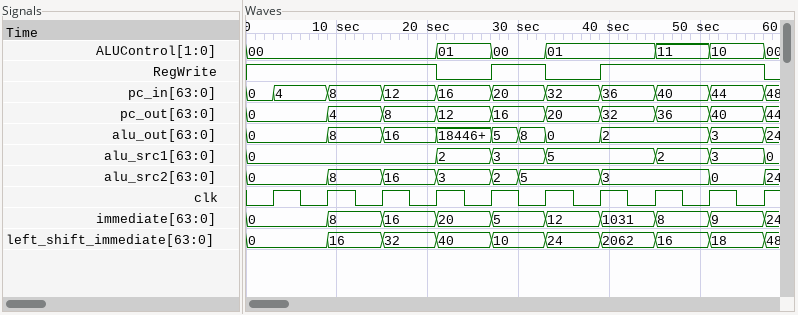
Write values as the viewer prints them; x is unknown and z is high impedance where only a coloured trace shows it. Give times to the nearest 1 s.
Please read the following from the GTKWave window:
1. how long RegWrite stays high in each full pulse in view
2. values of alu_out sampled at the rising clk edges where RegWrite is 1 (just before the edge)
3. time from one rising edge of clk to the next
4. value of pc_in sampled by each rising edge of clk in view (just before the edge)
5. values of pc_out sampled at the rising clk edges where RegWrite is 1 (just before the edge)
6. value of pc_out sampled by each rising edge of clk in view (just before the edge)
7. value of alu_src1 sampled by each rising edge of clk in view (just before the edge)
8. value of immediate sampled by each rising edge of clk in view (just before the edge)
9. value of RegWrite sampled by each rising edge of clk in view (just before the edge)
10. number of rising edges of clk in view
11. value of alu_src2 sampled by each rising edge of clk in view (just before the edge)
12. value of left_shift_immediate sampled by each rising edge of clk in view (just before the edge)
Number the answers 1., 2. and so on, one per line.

1. 6 s, 18 s
2. 0, 0, 8, 16, 8, 2, 2, 3
3. 6 s
4. 0, 4, 8, 12, 16, 20, 32, 36, 40, 44
5. 0, 0, 4, 8, 16, 32, 36, 40
6. 0, 0, 4, 8, 12, 16, 20, 32, 36, 40
7. 0, 0, 0, 0, 2, 3, 5, 5, 2, 3
8. 0, 0, 8, 16, 20, 5, 12, 1031, 8, 9
9. 1 1 1 1 0 1 0 1 1 1
10. 10
11. 0, 0, 8, 16, 3, 5, 5, 3, 3, 0
12. 0, 0, 16, 32, 40, 10, 24, 2062, 16, 18
